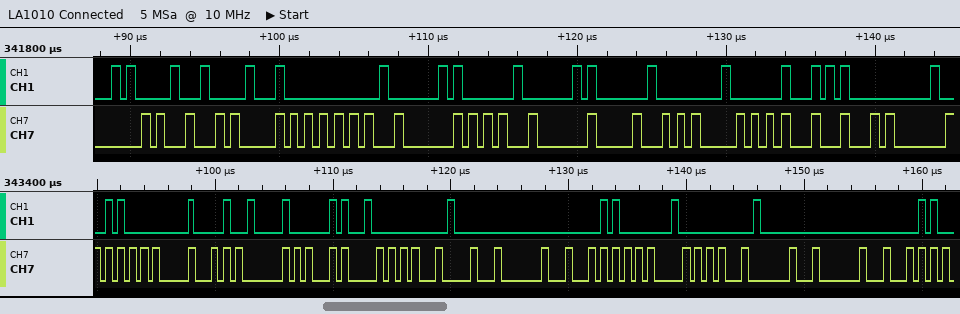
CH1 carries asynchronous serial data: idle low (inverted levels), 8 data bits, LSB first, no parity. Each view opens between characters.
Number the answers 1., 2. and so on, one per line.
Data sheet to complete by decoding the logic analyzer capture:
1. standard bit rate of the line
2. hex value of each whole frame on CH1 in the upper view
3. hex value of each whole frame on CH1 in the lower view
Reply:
1. 2000000 baud
2. 7D, DF, FF, 7F, 7F, FD, FF, 7F, F5
3. FD, DF, DF, DD, FF, FD, FF, FF
